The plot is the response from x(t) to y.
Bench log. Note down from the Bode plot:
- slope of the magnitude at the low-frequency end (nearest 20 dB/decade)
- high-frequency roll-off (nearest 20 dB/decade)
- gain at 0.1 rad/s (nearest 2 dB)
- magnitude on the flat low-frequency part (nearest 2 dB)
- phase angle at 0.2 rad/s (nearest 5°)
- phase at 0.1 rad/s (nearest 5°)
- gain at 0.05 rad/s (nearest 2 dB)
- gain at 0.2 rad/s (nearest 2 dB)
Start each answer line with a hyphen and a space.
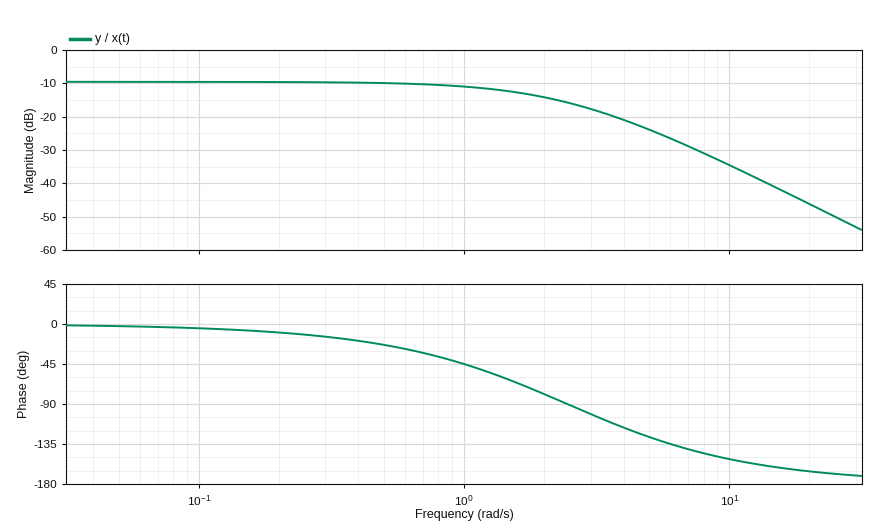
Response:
- 0 dB/decade
- -40 dB/decade
- -10 dB
- -10 dB
- -10°
- -5°
- -10 dB
- -10 dB
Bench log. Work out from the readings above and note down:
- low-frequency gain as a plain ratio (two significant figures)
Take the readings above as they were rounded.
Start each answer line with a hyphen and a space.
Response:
- 0.32
